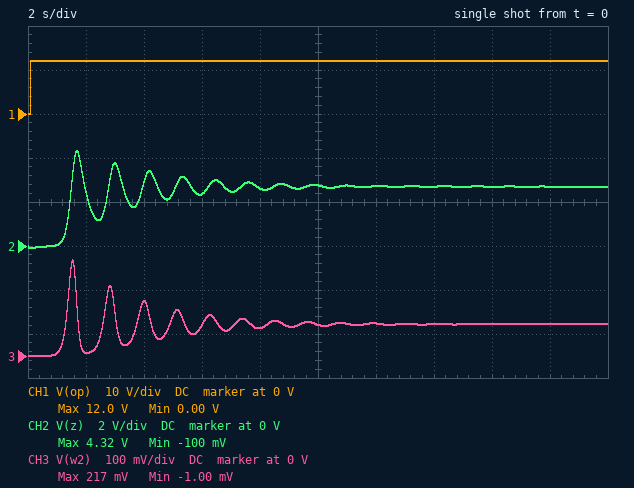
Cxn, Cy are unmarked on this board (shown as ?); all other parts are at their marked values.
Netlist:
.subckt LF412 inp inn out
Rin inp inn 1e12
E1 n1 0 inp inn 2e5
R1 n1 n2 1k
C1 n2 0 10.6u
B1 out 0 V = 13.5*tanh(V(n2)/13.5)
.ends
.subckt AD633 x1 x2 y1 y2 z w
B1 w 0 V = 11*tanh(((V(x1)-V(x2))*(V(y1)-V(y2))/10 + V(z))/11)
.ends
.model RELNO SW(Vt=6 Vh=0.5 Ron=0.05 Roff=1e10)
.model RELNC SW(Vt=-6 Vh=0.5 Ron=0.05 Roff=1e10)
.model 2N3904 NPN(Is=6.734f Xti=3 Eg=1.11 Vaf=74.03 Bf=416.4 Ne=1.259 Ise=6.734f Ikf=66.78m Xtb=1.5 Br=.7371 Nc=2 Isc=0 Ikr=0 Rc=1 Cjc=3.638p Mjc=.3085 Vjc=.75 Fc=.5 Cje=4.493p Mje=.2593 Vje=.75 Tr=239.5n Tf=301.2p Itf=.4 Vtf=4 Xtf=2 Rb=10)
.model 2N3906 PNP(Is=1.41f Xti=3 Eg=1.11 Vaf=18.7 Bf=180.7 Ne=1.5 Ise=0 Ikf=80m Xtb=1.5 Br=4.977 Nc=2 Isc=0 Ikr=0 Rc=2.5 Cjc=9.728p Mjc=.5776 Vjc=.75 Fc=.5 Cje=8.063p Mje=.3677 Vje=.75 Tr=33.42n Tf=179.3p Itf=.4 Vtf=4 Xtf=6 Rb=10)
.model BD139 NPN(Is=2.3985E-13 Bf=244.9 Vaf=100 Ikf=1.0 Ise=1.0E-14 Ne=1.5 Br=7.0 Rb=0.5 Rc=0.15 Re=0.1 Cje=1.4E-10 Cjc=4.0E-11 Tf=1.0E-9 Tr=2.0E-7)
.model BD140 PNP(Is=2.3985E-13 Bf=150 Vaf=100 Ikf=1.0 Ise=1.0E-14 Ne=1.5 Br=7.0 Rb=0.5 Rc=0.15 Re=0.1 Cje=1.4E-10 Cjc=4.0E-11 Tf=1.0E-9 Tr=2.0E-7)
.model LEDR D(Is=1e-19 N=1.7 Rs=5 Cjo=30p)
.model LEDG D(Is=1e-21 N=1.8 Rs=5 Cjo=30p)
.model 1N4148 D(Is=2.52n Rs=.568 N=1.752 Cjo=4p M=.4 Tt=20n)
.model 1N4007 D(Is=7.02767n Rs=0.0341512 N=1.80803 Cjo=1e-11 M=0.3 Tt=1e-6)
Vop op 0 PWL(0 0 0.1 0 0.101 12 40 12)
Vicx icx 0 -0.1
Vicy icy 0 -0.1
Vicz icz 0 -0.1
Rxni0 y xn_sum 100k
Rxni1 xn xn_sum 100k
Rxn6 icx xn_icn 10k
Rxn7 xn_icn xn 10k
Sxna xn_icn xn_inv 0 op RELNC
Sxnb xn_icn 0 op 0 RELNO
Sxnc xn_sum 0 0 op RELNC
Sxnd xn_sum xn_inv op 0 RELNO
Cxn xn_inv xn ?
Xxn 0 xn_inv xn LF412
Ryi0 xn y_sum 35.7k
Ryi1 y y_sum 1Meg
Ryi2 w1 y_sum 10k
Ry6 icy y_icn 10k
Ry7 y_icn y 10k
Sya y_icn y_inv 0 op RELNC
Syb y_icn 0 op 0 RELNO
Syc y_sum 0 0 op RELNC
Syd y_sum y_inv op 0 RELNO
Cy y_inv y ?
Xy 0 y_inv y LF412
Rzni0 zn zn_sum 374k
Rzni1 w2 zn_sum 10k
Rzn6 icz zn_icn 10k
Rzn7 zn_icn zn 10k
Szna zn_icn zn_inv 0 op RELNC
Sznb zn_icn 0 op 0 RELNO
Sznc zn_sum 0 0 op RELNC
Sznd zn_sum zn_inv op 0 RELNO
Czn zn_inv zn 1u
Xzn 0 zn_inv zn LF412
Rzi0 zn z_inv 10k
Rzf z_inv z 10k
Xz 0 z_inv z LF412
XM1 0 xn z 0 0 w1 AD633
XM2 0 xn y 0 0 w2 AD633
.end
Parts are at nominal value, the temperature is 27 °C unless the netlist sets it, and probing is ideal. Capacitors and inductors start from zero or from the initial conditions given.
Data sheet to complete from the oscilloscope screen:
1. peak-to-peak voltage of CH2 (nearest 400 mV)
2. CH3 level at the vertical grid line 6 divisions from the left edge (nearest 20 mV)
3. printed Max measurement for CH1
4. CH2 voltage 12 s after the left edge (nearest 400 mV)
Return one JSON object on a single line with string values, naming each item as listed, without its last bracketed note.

{"peak-to-peak voltage of CH2": "4.4 V", "CH3 level at the vertical grid line 6 divisions from the left edge": "80 mV", "printed Max measurement for CH1": "12.0 V", "CH2 voltage 12 s after the left edge": "2.8 V"}
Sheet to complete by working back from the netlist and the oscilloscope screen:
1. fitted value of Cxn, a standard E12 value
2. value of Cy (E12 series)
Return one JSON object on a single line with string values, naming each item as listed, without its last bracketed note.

{"fitted value of Cxn, a standard E12 value": "1.8 µF", "value of Cy": "3.3 µF"}
